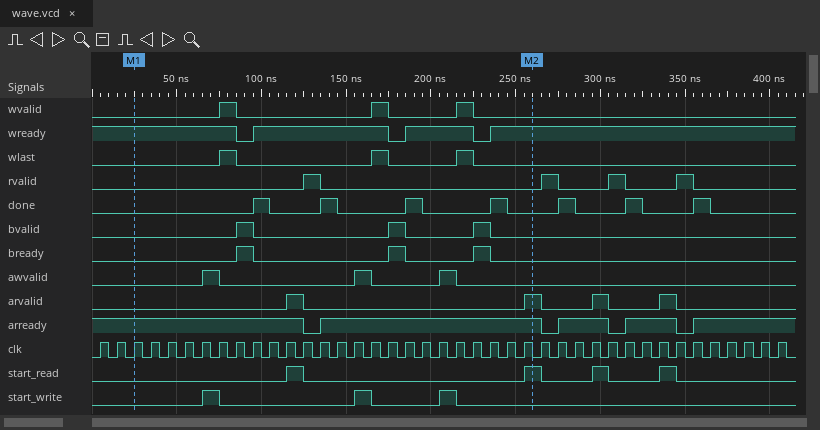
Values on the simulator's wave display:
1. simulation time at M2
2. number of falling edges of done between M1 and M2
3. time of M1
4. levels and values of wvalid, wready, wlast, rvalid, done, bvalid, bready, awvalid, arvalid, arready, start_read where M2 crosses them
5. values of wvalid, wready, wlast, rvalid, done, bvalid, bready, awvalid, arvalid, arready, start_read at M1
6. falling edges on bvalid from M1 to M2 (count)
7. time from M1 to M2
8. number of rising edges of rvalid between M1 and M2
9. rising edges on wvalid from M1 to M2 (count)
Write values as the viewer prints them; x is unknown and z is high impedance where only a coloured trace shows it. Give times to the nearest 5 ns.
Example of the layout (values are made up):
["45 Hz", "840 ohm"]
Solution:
["260 ns", "4", "25 ns", "wvalid=0, wready=1, wlast=0, rvalid=0, done=0, bvalid=0, bready=0, awvalid=0, arvalid=1, arready=1, start_read=1", "wvalid=0, wready=1, wlast=0, rvalid=0, done=0, bvalid=0, bready=0, awvalid=0, arvalid=0, arready=1, start_read=0", "3", "235 ns", "1", "3"]
